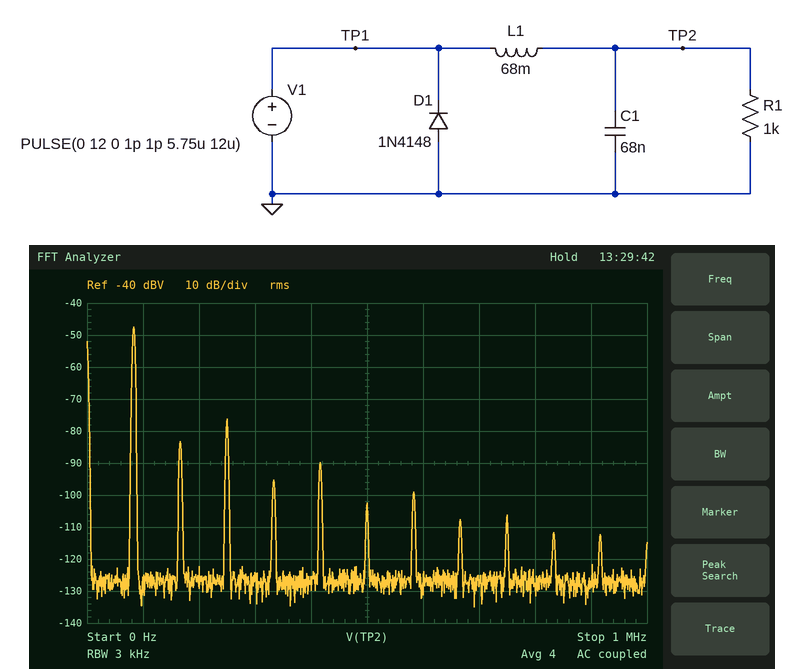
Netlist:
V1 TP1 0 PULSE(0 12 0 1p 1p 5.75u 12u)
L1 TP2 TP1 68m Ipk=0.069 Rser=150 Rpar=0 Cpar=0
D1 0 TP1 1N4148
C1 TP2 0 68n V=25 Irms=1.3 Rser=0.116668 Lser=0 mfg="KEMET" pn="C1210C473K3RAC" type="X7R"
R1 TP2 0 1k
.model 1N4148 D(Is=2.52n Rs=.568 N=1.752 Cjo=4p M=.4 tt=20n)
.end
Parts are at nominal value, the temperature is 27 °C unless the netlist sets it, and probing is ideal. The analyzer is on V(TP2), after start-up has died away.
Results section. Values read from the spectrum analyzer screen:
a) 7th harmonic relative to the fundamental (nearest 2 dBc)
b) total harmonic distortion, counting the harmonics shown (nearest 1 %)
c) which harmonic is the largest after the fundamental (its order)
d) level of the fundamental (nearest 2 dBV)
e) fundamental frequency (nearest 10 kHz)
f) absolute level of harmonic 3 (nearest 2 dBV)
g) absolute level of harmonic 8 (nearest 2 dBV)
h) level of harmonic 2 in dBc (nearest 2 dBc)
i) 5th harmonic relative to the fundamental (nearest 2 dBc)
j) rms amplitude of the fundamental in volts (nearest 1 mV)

-52 dBc
4 %
3
-48 dBV
80 kHz
-76 dBV
-108 dBV
-36 dBc
-42 dBc
4 mV
